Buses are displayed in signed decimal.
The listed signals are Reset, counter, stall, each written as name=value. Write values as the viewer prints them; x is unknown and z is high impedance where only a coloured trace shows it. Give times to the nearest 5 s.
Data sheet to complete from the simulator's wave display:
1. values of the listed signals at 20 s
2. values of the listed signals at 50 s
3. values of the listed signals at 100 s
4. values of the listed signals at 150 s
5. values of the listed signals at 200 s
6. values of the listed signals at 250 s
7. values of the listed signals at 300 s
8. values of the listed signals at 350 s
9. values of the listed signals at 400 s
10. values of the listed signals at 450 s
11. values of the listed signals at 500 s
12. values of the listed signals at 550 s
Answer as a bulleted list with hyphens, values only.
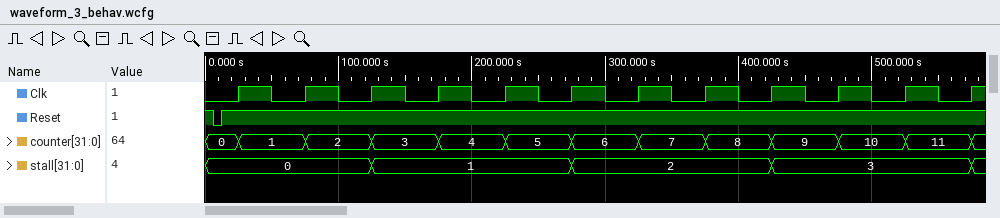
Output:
- Reset=1, counter=0, stall=0
- Reset=1, counter=1, stall=0
- Reset=1, counter=2, stall=0
- Reset=1, counter=3, stall=1
- Reset=1, counter=4, stall=1
- Reset=1, counter=5, stall=1
- Reset=1, counter=6, stall=2
- Reset=1, counter=7, stall=2
- Reset=1, counter=8, stall=2
- Reset=1, counter=9, stall=3
- Reset=1, counter=10, stall=3
- Reset=1, counter=11, stall=3
